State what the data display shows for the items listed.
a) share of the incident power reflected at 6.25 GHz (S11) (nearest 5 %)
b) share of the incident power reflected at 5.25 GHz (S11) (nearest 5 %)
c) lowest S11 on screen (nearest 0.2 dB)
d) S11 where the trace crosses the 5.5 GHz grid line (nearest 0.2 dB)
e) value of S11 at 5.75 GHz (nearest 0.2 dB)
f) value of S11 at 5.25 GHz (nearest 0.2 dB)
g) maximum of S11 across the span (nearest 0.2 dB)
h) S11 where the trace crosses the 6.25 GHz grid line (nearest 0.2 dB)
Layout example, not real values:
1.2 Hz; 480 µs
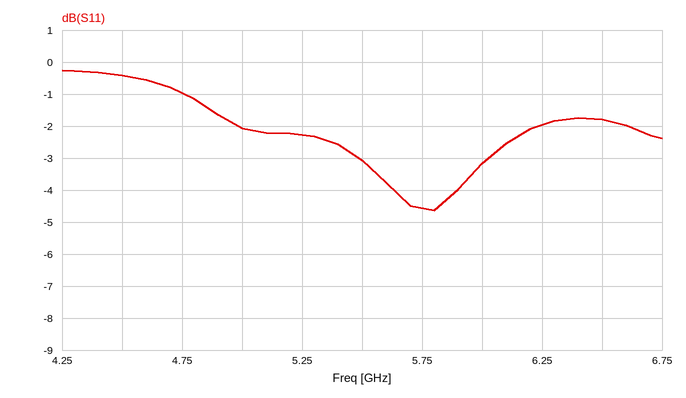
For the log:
65 %; 60 %; -4.6 dB; -3.0 dB; -4.6 dB; -2.2 dB; -0.2 dB; -2.0 dB
